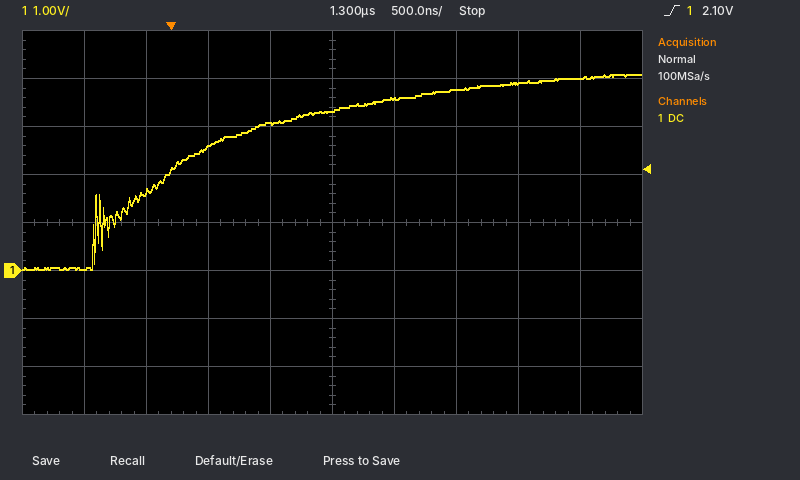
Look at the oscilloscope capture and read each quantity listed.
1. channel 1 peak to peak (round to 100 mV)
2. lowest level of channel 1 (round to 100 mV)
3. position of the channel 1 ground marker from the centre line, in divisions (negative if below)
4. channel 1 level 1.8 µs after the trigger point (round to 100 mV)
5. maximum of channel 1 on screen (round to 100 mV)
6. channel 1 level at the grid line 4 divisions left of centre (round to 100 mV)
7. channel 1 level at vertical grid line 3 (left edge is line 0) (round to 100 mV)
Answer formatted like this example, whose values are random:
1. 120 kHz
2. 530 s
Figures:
1. 4.1 V
2. 0.0 V
3. -1.0 div
4. 3.6 V
5. 4.1 V
6. 0.0 V
7. 2.6 V
